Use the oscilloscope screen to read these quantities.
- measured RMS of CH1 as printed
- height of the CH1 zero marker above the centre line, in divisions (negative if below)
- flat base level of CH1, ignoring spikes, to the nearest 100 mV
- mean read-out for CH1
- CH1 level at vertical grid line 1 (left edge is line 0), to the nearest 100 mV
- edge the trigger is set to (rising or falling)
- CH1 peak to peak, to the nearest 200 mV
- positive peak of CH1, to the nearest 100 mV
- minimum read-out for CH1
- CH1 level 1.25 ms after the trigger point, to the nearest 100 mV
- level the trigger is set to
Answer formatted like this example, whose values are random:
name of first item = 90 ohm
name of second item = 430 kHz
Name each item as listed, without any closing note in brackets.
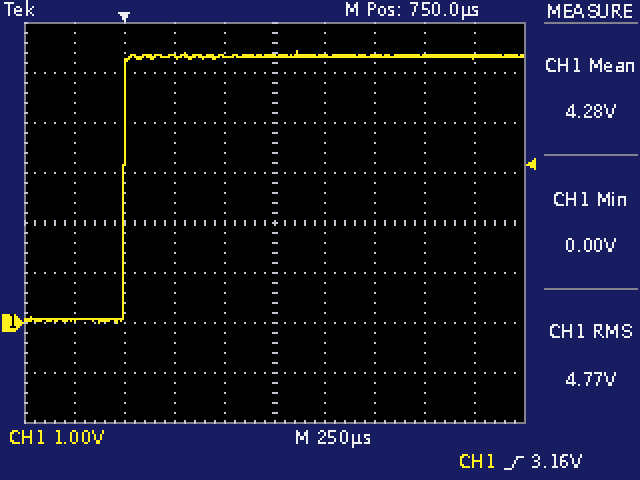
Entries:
measured RMS of CH1 as printed = 4.77 V
height of the CH1 zero marker above the centre line, in divisions = -2.0 div
flat base level of CH1, ignoring spikes, to the nearest 100 mV = 100 mV
mean read-out for CH1 = 4.28 V
CH1 level at vertical grid line 1 (left edge is line 0), to the nearest 100 mV = 100 mV
edge the trigger is set to = rising
CH1 peak to peak, to the nearest 200 mV = 5.4 V
positive peak of CH1, to the nearest 100 mV = 5.4 V
minimum read-out for CH1 = 0.00 V
CH1 level 1.25 ms after the trigger point, to the nearest 100 mV = 5.3 V
level the trigger is set to = 3.16 V
